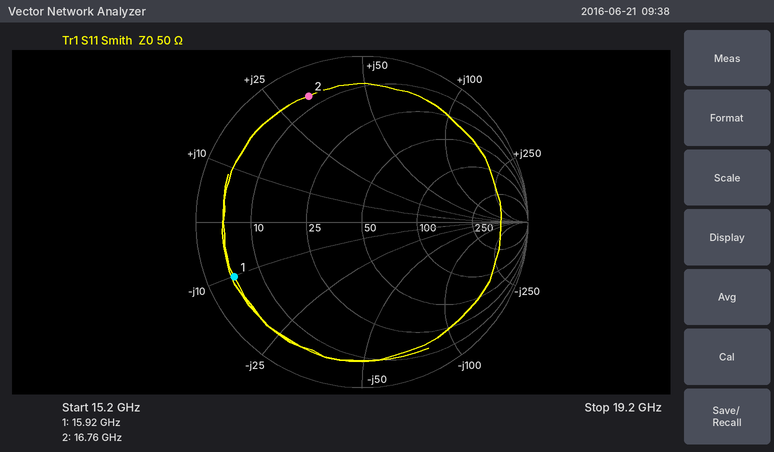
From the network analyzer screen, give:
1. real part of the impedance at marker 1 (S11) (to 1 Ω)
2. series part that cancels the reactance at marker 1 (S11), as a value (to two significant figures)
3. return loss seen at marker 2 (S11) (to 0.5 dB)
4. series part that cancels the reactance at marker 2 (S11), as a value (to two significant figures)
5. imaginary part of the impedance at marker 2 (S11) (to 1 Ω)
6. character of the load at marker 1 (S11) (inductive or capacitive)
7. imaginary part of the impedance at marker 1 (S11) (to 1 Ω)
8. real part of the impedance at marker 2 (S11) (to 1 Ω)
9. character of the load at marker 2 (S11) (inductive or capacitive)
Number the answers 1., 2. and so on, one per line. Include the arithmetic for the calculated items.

1. 5 Ω
2. L = 10 Ω/(2π × 15.92 GHz) ≈ 100 pH
3. 1.5 dB
4. C = 1/(2π × 16.76 GHz × 33 Ω) ≈ 288 fF, so 290 fF to two significant figures
5. +33 Ω
6. capacitive
7. -10 Ω
8. 7 Ω
9. inductive
